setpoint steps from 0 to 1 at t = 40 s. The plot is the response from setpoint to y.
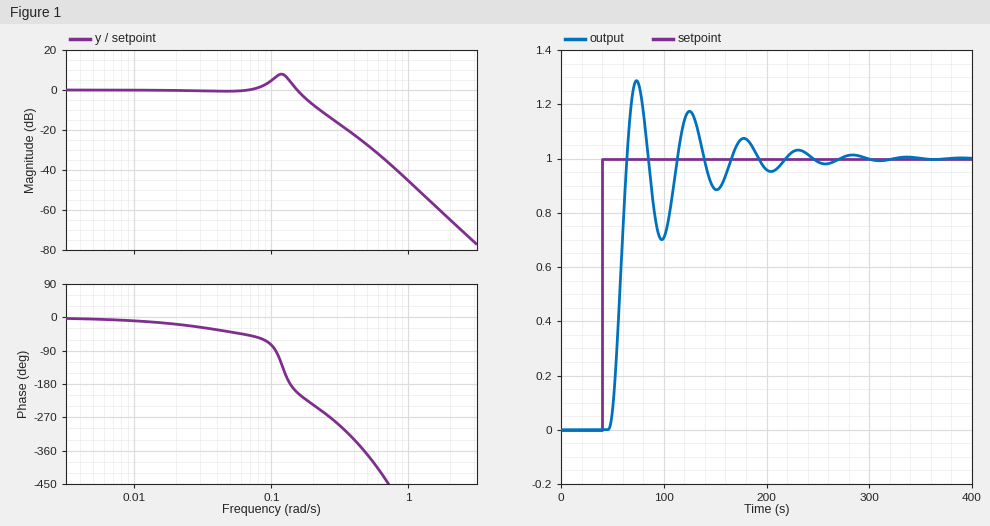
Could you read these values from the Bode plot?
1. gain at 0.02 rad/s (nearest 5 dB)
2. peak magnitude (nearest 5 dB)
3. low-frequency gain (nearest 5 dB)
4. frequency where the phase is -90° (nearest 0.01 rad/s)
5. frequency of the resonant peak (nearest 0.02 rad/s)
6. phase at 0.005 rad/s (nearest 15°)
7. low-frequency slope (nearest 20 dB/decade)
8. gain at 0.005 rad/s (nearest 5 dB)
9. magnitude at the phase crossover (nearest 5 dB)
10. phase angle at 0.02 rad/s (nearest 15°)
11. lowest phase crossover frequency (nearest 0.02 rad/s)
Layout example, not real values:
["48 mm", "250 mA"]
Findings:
["0 dB", "10 dB", "0 dB", "0.11 rad/s", "0.12 rad/s", "0°", "0 dB/decade", "0 dB", "5 dB", "-15°", "0.14 rad/s"]
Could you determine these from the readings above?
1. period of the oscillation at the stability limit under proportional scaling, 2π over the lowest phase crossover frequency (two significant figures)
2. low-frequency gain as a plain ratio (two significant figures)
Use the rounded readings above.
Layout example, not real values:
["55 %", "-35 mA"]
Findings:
["45 s", "1.0"]
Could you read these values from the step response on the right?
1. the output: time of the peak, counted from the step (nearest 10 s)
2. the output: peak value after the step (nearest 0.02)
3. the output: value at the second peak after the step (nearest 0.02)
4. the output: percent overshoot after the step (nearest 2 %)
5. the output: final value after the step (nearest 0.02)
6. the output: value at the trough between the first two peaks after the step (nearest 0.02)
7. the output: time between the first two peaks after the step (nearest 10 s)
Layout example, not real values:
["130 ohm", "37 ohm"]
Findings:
["30 s", "1.28", "1.18", "28 %", "1.00", "0.70", "50 s"]
